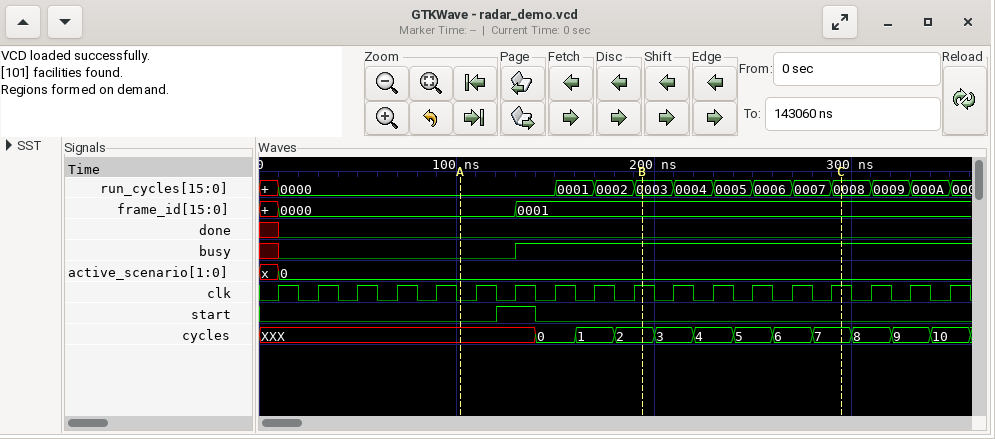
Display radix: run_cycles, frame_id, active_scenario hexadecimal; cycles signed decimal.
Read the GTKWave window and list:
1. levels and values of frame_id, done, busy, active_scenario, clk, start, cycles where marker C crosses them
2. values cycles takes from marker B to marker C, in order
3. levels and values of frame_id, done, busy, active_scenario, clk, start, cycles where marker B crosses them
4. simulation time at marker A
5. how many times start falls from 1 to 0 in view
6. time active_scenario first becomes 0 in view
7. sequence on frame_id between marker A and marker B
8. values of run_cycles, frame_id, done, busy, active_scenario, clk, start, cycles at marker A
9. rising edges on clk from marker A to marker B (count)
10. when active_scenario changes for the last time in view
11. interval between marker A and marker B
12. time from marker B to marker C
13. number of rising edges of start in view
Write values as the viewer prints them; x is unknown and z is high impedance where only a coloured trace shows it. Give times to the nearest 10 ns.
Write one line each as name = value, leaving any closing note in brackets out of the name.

levels and values of frame_id, done, busy, active_scenario, clk, start, cycles where marker C crosses them = frame_id=0001, done=0, busy=1, active_scenario=0, clk=1, start=0, cycles=7
values cycles takes from marker B to marker C, in order = 2, 3, 4, 5, 6, 7
levels and values of frame_id, done, busy, active_scenario, clk, start, cycles where marker B crosses them = frame_id=0001, done=0, busy=1, active_scenario=0, clk=1, start=0, cycles=2
simulation time at marker A = 100 ns
how many times start falls from 1 to 0 in view = 1
time active_scenario first becomes 0 in view = 10 ns
sequence on frame_id between marker A and marker B = 0000, 0001
values of run_cycles, frame_id, done, busy, active_scenario, clk, start, cycles at marker A = run_cycles=0000, frame_id=0000, done=0, busy=0, active_scenario=0, clk=0, start=0, cycles=XXX
rising edges on clk from marker A to marker B = 5
when active_scenario changes for the last time in view = 10 ns
interval between marker A and marker B = 90 ns
time from marker B to marker C = 100 ns
number of rising edges of start in view = 1
